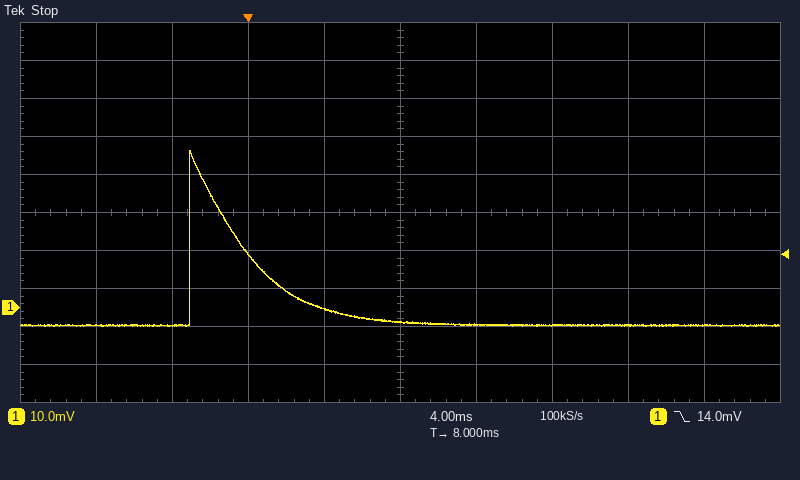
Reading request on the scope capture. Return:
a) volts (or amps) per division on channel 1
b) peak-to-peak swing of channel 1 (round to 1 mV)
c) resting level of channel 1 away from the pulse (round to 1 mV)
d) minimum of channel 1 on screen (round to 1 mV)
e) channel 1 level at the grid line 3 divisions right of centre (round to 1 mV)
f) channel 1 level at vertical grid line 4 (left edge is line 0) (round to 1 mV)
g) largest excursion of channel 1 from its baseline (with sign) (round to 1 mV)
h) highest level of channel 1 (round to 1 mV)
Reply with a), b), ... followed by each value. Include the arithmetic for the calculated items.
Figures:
a) 10 mV
b) 41 mV − (-5 mV) = 46 mV
c) -5 mV
d) -5 mV
e) -5 mV
f) 0 mV
g) 41 mV − (-5 mV) = +46 mV
h) 41 mV
